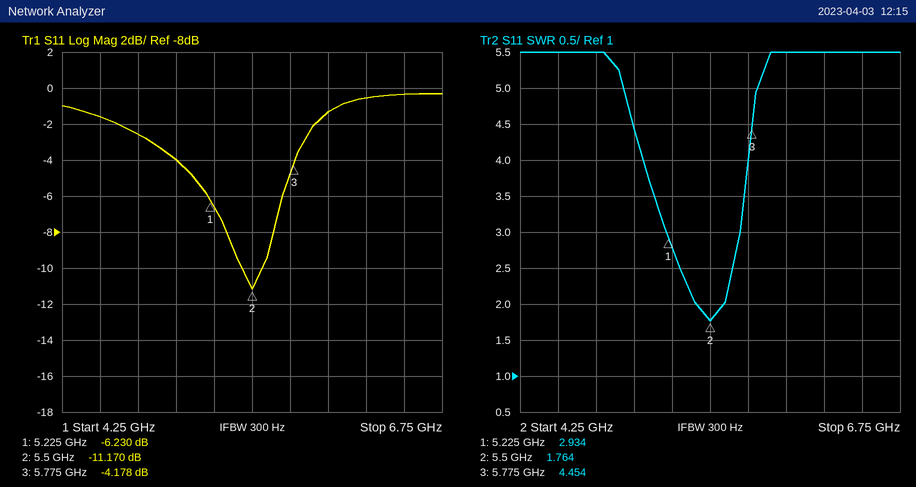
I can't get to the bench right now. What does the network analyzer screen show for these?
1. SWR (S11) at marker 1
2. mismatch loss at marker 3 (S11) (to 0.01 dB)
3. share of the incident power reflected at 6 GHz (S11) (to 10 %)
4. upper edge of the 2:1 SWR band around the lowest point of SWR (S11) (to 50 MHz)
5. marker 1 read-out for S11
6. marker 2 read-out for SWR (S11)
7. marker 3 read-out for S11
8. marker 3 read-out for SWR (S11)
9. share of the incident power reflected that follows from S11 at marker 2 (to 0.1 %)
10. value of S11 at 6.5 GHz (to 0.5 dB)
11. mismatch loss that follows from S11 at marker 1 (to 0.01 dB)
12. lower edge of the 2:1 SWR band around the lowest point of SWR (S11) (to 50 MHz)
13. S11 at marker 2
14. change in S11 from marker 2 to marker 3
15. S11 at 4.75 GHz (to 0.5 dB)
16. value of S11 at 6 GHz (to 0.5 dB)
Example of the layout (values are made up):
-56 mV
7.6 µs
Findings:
2.934
2.09 dB
70 %
5.60 GHz
-6.230 dB
1.764
-4.178 dB
4.454
7.6 %
-0.5 dB
1.18 dB
5.40 GHz
-11.170 dB
6.992 dB
-2.5 dB
-1.5 dB
